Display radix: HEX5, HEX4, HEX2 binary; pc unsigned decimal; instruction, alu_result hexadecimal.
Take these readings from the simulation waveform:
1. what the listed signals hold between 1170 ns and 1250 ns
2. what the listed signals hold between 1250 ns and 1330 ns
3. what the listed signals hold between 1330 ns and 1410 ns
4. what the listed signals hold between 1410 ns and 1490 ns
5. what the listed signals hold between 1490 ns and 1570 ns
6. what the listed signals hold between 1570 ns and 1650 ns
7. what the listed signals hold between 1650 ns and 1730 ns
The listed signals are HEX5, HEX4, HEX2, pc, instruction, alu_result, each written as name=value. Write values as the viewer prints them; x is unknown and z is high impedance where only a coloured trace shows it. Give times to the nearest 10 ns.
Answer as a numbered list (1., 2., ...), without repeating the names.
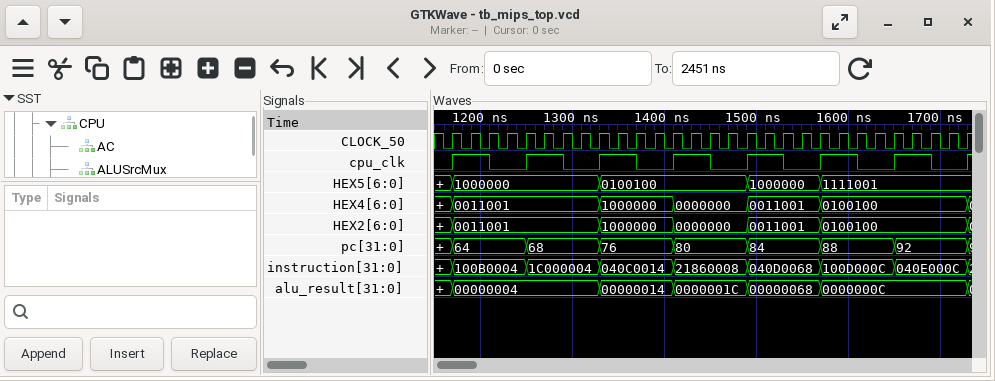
1. HEX5=1000000, HEX4=0011001, HEX2=0011001, pc=64, instruction=100B0004, alu_result=00000004
2. HEX5=1000000, HEX4=0011001, HEX2=0011001, pc=68, instruction=1C000004, alu_result=00000004
3. HEX5=0100100, HEX4=1000000, HEX2=1000000, pc=76, instruction=040C0014, alu_result=00000014
4. HEX5=0100100, HEX4=0000000, HEX2=0000000, pc=80, instruction=21860008, alu_result=0000001C
5. HEX5=1000000, HEX4=0011001, HEX2=0011001, pc=84, instruction=040D0068, alu_result=00000068
6. HEX5=1111001, HEX4=0100100, HEX2=0100100, pc=88, instruction=100D000C, alu_result=0000000C
7. HEX5=1111001, HEX4=0100100, HEX2=0100100, pc=92, instruction=040E000C, alu_result=0000000C
